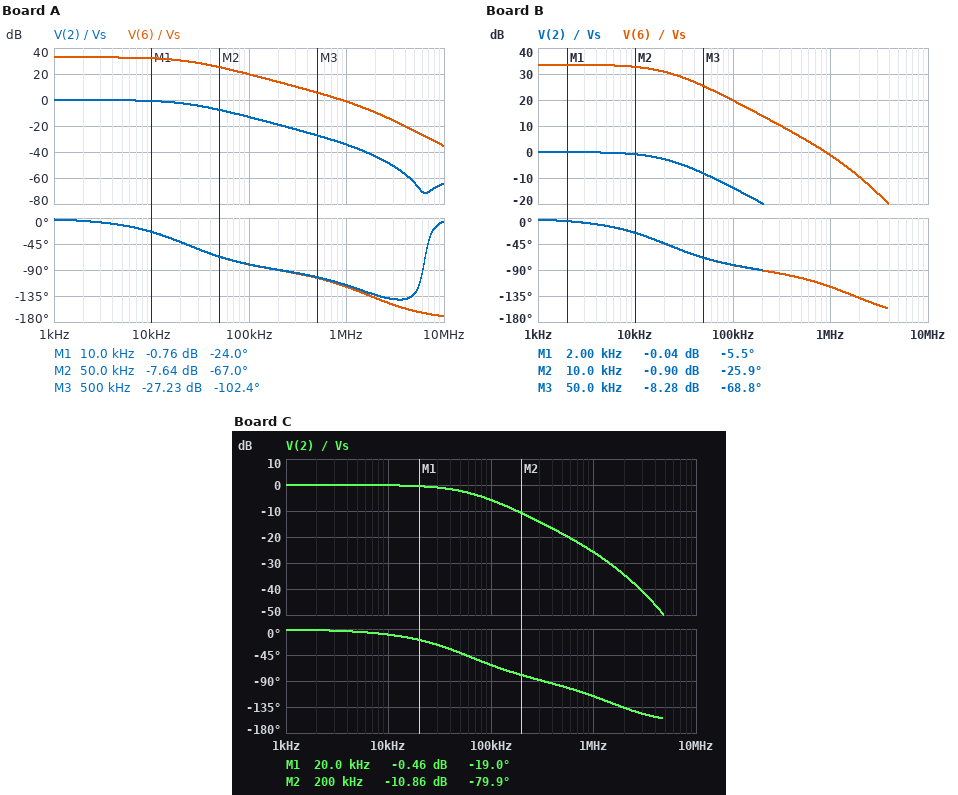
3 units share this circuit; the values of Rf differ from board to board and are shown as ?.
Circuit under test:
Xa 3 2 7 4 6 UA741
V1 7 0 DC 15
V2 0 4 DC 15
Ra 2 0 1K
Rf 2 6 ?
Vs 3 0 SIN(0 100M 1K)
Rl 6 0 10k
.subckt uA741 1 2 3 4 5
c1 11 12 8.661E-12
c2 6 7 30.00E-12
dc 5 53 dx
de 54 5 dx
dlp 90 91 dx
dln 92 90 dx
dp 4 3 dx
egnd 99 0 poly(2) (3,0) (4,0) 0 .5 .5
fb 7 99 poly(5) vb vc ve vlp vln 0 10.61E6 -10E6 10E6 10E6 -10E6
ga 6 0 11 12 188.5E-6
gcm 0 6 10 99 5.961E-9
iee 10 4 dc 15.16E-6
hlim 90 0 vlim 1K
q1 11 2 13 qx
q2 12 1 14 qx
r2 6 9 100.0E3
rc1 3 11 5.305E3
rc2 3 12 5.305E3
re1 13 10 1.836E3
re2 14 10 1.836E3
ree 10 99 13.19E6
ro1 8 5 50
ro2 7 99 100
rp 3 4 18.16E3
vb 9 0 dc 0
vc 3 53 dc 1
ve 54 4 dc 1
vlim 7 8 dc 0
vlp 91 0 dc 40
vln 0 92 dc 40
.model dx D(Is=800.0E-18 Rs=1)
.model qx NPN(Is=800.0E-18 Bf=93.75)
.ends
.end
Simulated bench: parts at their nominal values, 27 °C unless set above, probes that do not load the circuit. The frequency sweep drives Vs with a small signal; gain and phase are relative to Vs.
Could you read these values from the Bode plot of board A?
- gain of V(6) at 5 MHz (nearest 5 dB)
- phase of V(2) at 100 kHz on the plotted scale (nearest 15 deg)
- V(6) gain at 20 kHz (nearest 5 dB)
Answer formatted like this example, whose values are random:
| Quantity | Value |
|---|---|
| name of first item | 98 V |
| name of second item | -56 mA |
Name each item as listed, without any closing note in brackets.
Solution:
| Quantity | Value |
|---|---|
| gain of V(6) at 5 MHz | -25 dB |
| phase of V(2) at 100 kHz on the plotted scale | -75 deg |
| V(6) gain at 20 kHz | 30 dB |
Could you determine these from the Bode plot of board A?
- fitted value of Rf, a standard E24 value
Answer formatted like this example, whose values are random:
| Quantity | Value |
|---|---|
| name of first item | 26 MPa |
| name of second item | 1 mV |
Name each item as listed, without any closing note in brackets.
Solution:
| Quantity | Value |
|---|---|
| fitted value of Rf, a standard E24 value | 43 kΩ |
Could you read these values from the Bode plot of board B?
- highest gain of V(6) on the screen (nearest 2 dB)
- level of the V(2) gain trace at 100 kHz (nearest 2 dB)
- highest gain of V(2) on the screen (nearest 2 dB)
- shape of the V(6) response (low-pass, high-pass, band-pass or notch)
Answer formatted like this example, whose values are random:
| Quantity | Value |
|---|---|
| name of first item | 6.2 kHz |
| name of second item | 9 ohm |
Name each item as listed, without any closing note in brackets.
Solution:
| Quantity | Value |
|---|---|
| highest gain of V(6) on the screen | 34 dB |
| level of the V(2) gain trace at 100 kHz | -14 dB |
| highest gain of V(2) on the screen | 0 dB |
| shape of the V(6) response | low-pass |
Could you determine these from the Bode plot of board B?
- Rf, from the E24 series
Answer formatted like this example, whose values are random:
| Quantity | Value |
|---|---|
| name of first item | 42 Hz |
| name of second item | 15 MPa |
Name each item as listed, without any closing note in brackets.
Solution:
| Quantity | Value |
|---|---|
| Rf, from the E24 series | 47 kΩ |
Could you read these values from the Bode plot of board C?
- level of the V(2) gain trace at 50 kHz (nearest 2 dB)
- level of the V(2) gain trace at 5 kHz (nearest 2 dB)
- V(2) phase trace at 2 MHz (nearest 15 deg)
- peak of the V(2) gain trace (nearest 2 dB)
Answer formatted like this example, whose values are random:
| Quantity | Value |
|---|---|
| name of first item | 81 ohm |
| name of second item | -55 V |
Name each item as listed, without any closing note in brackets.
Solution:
| Quantity | Value |
|---|---|
| level of the V(2) gain trace at 50 kHz | -2 dB |
| level of the V(2) gain trace at 5 kHz | 0 dB |
| V(2) phase trace at 2 MHz | -135 deg |
| peak of the V(2) gain trace | 0 dB |
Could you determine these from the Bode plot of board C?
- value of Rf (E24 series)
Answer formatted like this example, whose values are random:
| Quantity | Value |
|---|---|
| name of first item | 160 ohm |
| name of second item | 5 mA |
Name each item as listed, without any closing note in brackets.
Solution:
| Quantity | Value |
|---|---|
| value of Rf | 16 kΩ |
